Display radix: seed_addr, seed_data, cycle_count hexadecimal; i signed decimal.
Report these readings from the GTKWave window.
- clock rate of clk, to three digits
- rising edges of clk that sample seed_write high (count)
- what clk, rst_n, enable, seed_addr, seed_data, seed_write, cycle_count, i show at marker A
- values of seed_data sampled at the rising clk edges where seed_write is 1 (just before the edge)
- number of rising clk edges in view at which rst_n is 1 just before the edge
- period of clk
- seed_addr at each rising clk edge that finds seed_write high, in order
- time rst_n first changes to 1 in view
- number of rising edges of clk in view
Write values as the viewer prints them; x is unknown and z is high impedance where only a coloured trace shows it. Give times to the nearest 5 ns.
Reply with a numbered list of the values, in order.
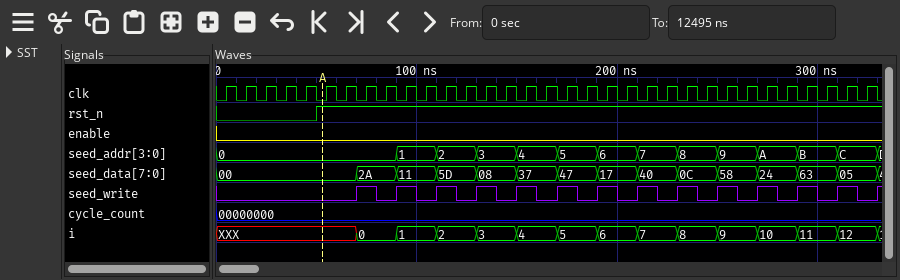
1. 100 MHz
2. 13
3. clk=0, rst_n=1, enable=0, seed_addr=0, seed_data=00, seed_write=0, cycle_count=00000000, i=XXX
4. 2A, 11, 5D, 08, 37, 47, 17, 40, 0C, 58, 24, 63, 05
5. 28
6. 10 ns
7. 0, 1, 2, 3, 4, 5, 6, 7, 8, 9, A, B, C
8. 50 ns
9. 33
